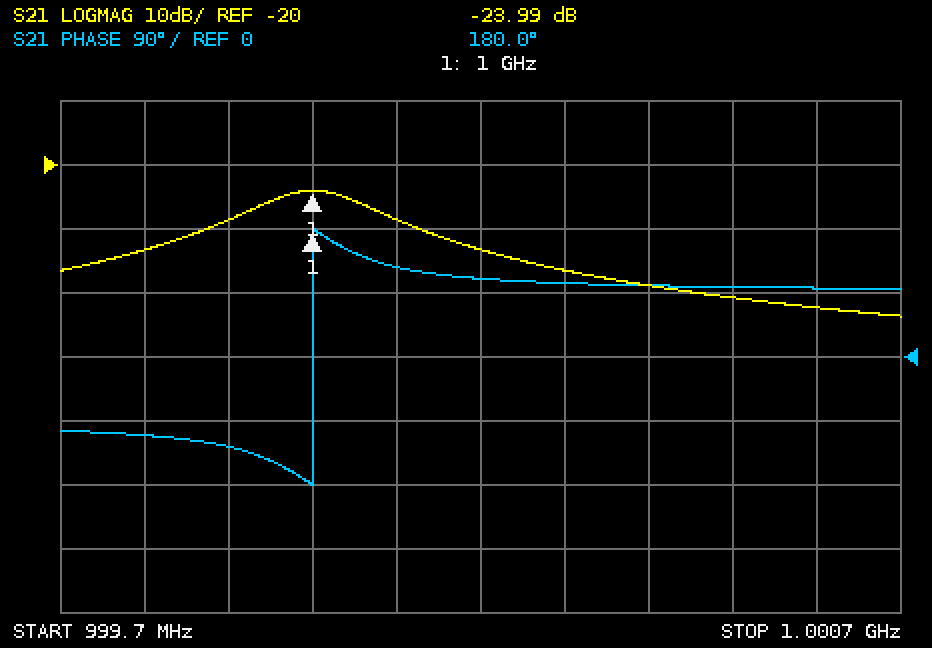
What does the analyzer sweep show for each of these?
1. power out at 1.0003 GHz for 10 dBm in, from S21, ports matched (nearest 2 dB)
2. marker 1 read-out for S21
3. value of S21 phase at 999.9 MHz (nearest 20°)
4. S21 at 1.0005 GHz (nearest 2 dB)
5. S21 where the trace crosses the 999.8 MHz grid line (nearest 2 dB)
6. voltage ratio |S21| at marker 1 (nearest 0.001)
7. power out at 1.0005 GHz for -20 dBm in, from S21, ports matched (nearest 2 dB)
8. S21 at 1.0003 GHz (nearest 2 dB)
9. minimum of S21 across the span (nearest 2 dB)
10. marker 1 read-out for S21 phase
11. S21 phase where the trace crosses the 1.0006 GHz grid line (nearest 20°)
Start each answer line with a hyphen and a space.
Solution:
- -26 dBm
- -23.99 dB
- -120°
- -40 dB
- -34 dB
- 0.063
- -60 dBm
- -36 dB
- -44 dB
- 180.0°
- 100°
